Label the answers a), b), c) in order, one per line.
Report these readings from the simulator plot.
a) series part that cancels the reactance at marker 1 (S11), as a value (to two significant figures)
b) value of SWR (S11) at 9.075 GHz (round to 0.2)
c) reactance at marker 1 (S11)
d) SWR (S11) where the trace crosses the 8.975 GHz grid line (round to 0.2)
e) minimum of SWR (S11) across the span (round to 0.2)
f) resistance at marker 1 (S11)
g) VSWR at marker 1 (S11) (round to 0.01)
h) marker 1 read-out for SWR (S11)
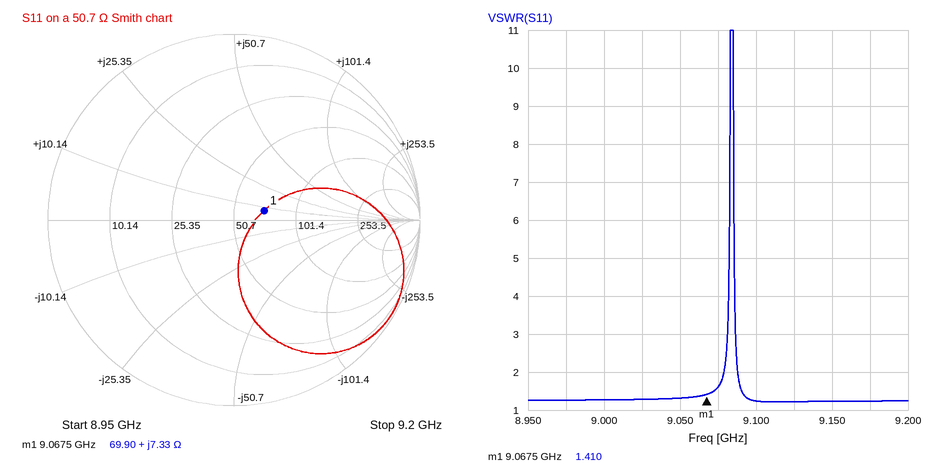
a) 2.4 pF
b) 1.6
c) +7.33 Ω
d) 1.2
e) 1.2
f) 69.90 Ω
g) 1.41
h) 1.410
